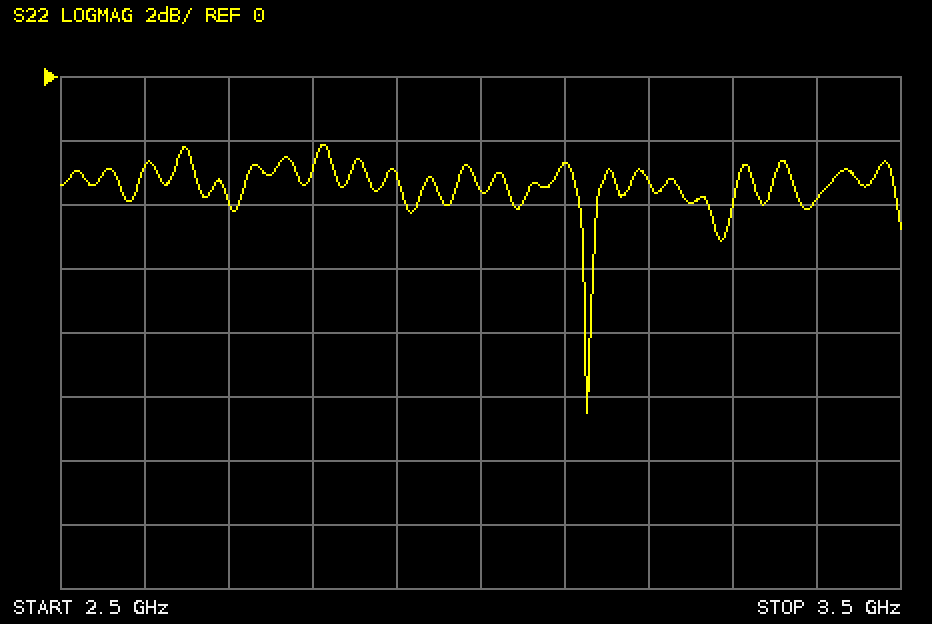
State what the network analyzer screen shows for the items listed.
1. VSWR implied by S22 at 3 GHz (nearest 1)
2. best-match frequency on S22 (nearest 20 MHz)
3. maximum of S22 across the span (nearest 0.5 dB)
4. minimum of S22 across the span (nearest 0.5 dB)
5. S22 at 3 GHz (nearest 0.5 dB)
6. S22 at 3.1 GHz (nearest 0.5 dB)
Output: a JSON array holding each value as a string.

["5", "3.12 GHz", "-2.0 dB", "-10.5 dB", "-3.5 dB", "-2.5 dB"]
